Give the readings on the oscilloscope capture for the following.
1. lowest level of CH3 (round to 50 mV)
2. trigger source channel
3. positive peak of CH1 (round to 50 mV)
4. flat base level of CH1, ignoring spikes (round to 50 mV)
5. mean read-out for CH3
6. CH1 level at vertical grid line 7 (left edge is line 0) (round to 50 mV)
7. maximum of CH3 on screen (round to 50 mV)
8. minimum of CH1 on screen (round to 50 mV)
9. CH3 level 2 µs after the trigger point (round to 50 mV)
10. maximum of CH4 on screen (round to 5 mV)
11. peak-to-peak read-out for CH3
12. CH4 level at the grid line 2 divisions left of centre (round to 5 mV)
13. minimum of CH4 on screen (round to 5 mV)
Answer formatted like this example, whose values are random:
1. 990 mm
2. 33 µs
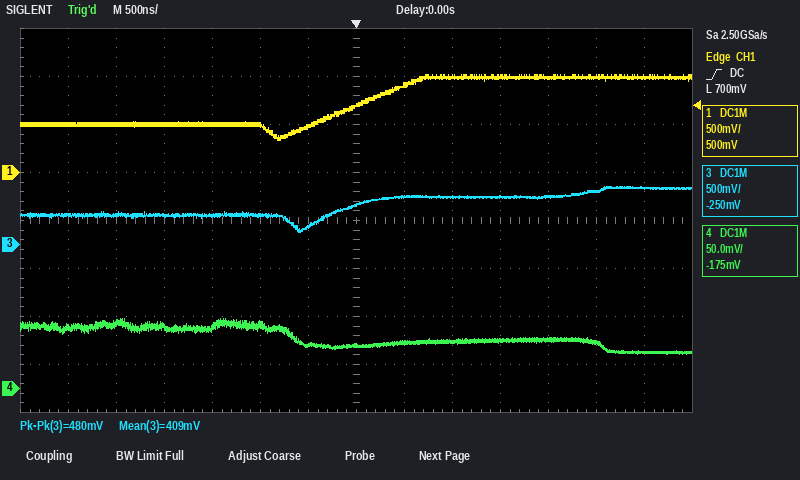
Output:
1. 100 mV
2. CH1
3. 1.00 V
4. 500 mV
5. 409 mV
6. 700 mV
7. 600 mV
8. 350 mV
9. 500 mV
10. 75 mV
11. 480 mV
12. 65 mV
13. 35 mV
